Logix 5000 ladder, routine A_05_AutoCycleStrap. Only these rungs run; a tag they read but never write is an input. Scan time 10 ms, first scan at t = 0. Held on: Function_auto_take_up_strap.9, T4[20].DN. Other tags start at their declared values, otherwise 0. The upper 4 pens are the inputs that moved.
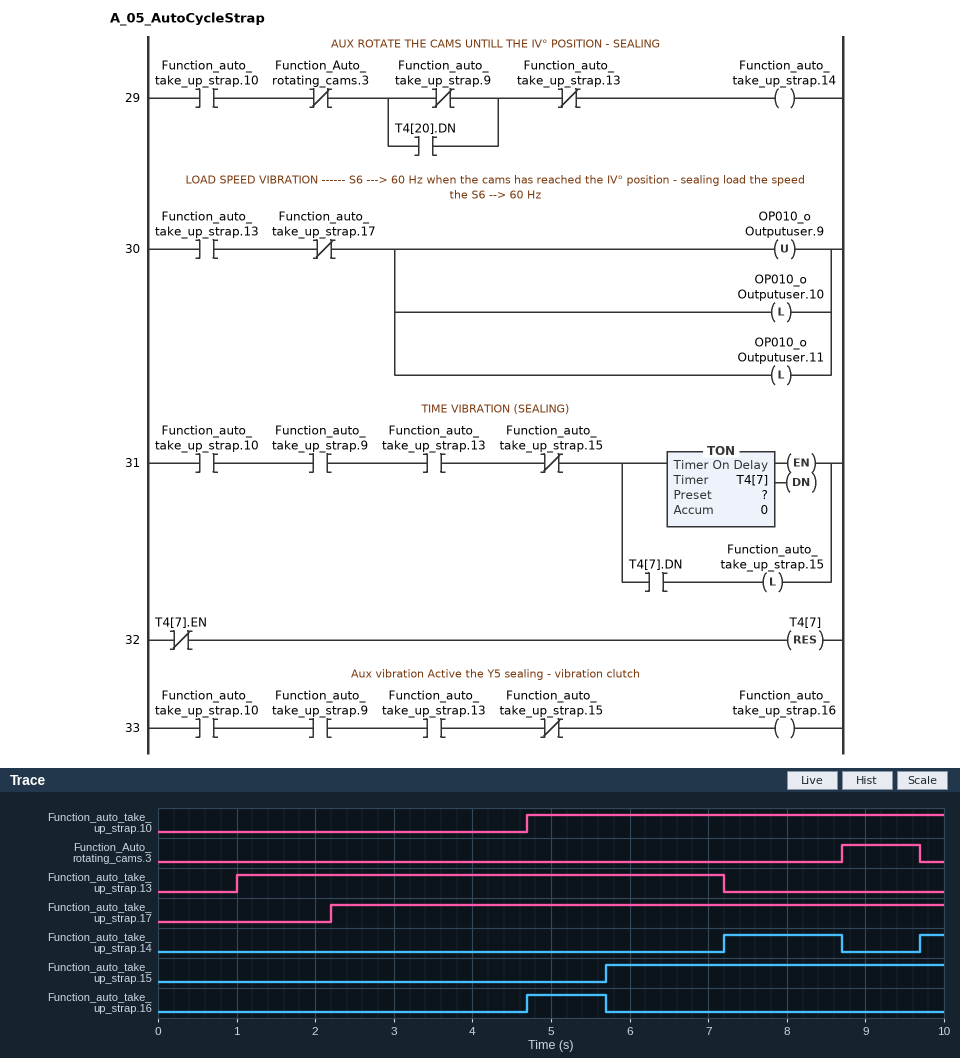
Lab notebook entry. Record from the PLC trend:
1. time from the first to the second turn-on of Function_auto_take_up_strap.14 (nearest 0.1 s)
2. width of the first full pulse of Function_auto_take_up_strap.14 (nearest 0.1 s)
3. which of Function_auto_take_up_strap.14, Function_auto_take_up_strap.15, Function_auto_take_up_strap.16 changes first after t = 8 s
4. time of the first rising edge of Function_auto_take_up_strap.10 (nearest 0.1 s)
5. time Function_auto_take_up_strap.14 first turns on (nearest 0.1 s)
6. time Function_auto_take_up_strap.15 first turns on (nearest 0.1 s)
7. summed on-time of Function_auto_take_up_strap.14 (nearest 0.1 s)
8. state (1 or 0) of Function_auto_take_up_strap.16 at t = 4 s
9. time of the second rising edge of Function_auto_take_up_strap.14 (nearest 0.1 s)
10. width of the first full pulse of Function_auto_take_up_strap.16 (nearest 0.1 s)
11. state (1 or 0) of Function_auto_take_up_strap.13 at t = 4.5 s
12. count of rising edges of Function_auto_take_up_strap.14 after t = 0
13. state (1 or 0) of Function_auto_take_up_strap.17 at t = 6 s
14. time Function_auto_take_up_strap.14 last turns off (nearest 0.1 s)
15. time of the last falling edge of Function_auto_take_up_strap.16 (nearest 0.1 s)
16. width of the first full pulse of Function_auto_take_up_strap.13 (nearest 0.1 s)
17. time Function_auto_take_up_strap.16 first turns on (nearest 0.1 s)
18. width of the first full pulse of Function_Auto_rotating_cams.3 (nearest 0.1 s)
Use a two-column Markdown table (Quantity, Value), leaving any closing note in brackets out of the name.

| Quantity | Value |
|---|---|
| time from the first to the second turn-on of Function_auto_take_up_strap.14 | 2.5 s |
| width of the first full pulse of Function_auto_take_up_strap.14 | 1.5 s |
| which of Function_auto_take_up_strap.14, Function_auto_take_up_strap.15, Function_auto_take_up_strap.16 changes first after t = 8 s | Function_auto_take_up_strap.14 |
| time of the first rising edge of Function_auto_take_up_strap.10 | 4.7 s |
| time Function_auto_take_up_strap.14 first turns on | 7.2 s |
| time Function_auto_take_up_strap.15 first turns on | 5.7 s |
| summed on-time of Function_auto_take_up_strap.14 | 1.8 s |
| state (1 or 0) of Function_auto_take_up_strap.16 at t = 4 s | 0 |
| time of the second rising edge of Function_auto_take_up_strap.14 | 9.7 s |
| width of the first full pulse of Function_auto_take_up_strap.16 | 1.0 s |
| state (1 or 0) of Function_auto_take_up_strap.13 at t = 4.5 s | 1 |
| count of rising edges of Function_auto_take_up_strap.14 after t = 0 | 2 |
| state (1 or 0) of Function_auto_take_up_strap.17 at t = 6 s | 1 |
| time Function_auto_take_up_strap.14 last turns off | 8.7 s |
| time of the last falling edge of Function_auto_take_up_strap.16 | 5.7 s |
| width of the first full pulse of Function_auto_take_up_strap.13 | 6.2 s |
| time Function_auto_take_up_strap.16 first turns on | 4.7 s |
| width of the first full pulse of Function_Auto_rotating_cams.3 | 1.0 s |
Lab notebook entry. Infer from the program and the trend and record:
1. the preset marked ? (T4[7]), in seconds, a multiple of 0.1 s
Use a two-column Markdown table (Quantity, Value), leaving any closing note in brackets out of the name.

| Quantity | Value |
|---|---|
| the preset marked ? (T4[7]), in seconds, a multiple of 0.1 s | 1.0 s |
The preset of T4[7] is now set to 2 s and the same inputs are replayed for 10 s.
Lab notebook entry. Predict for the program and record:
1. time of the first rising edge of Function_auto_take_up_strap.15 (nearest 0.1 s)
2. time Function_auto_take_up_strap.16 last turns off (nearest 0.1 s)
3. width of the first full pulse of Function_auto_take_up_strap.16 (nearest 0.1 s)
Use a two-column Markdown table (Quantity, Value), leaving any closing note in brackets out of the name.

| Quantity | Value |
|---|---|
| time of the first rising edge of Function_auto_take_up_strap.15 | 6.7 s |
| time Function_auto_take_up_strap.16 last turns off | 6.7 s |
| width of the first full pulse of Function_auto_take_up_strap.16 | 2.0 s |
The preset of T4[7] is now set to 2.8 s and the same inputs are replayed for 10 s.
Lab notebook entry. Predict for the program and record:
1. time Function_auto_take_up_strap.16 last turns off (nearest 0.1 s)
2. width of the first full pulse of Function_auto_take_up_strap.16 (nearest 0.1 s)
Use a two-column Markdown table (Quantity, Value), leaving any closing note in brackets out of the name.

| Quantity | Value |
|---|---|
| time Function_auto_take_up_strap.16 last turns off | 7.2 s |
| width of the first full pulse of Function_auto_take_up_strap.16 | 2.5 s |
